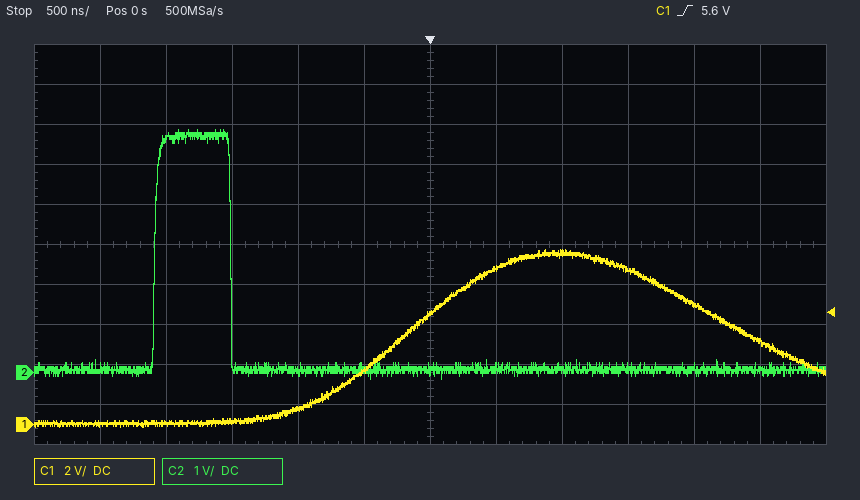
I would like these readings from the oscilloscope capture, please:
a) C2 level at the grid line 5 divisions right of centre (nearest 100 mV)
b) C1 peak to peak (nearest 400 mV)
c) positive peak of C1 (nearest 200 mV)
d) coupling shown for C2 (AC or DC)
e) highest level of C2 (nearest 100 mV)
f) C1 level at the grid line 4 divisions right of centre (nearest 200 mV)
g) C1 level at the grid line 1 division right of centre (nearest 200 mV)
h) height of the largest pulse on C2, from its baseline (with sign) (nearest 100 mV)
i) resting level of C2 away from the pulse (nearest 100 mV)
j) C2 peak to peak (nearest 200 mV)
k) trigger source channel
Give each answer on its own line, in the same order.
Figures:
100 mV
8.8 V
8.8 V
DC
6.1 V
6.0 V
7.8 V
+6.0 V
100 mV
6.2 V
C1
